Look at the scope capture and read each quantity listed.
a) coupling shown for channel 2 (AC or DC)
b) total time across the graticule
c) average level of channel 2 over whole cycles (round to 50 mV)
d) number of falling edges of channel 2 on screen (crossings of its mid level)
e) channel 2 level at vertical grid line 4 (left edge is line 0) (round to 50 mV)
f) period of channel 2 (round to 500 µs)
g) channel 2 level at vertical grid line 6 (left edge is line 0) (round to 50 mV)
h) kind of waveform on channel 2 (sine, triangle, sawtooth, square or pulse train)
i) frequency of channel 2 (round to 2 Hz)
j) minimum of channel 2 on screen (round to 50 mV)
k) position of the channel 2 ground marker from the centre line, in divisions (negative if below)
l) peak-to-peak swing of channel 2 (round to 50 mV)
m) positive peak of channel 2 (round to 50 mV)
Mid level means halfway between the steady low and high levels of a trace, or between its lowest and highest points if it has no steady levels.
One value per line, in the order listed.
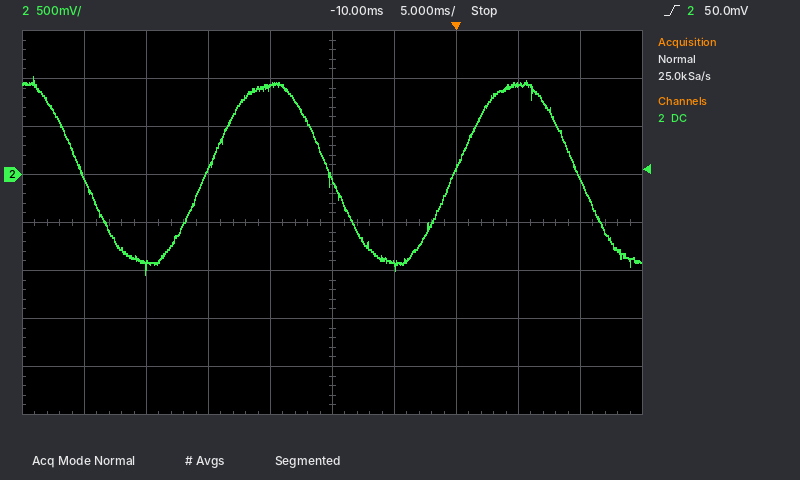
DC
50 ms
0 mV
3
900 mV
20.0 ms
-950 mV
sine
50 Hz
-1.05 V
+1.0 div
2.05 V
1.00 V
